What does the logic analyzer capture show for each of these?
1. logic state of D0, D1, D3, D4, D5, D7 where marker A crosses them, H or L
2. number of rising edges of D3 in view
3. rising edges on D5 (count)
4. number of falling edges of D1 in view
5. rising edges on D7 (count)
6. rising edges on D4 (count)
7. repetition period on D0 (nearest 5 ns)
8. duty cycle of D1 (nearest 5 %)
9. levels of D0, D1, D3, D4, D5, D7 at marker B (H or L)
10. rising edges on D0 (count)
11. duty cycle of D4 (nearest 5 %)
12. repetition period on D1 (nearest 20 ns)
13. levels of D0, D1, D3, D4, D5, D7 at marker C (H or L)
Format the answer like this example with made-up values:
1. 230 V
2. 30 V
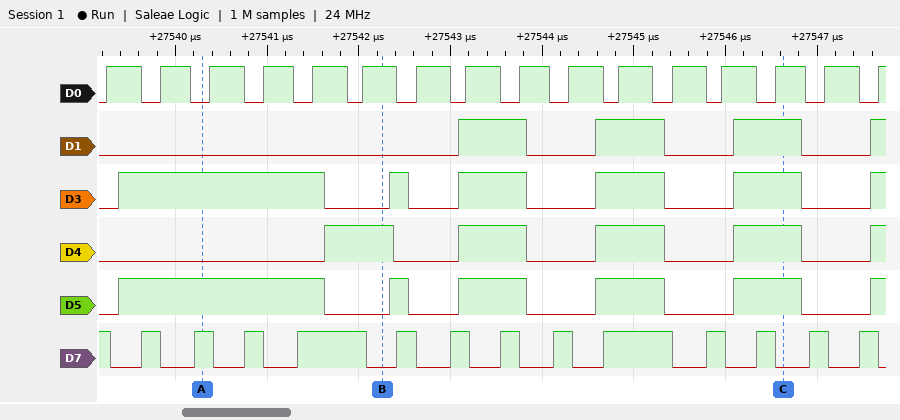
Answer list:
1. D0=L, D1=L, D3=H, D4=L, D5=H, D7=H
2. 6
3. 6
4. 3
5. 13
6. 5
7. 560 ns
8. 50 %
9. D0=H, D1=L, D3=L, D4=H, D5=L, D7=L
10. 16
11. 50 %
12. 1500 ns
13. D0=H, D1=H, D3=H, D4=H, D5=H, D7=L
